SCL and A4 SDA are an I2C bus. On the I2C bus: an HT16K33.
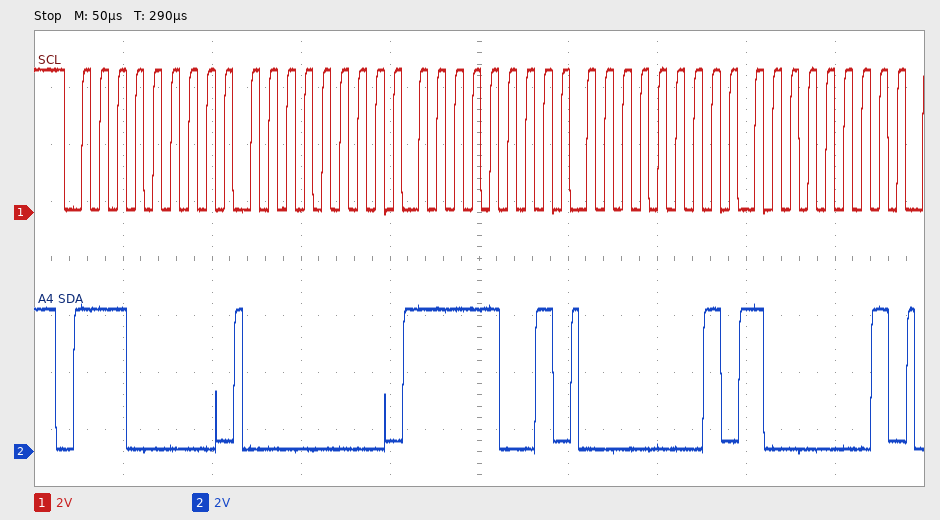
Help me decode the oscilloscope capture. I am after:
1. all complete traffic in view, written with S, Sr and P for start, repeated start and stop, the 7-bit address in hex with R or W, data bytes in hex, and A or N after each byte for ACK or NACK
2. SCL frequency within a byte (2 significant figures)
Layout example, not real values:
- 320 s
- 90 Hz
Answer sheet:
- S 70W A 00 A F9 A 01 A 81 A
- 100 kHz
